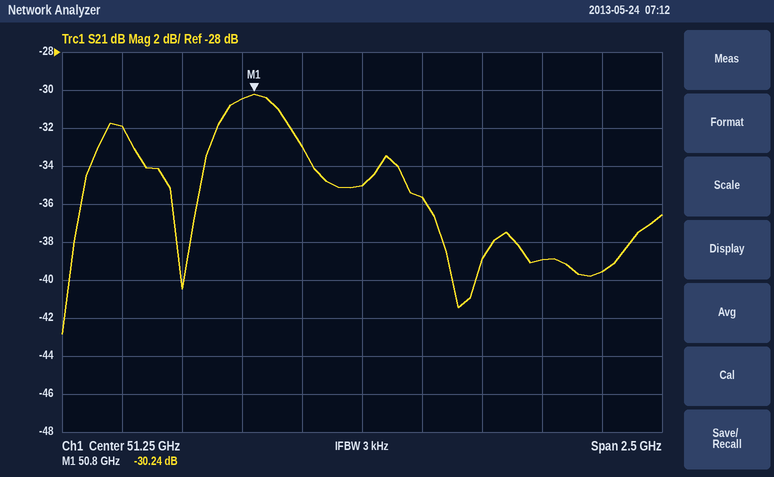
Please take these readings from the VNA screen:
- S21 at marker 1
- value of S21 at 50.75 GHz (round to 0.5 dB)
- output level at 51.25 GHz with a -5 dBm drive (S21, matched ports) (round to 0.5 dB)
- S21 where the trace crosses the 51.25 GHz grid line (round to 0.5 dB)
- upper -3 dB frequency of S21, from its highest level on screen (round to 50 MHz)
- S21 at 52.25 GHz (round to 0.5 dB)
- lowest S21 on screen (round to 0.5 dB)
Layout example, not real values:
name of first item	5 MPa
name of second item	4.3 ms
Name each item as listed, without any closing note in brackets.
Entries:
S21 at marker 1	-30.24 dB
value of S21 at 50.75 GHz	-30.5 dB
output level at 51.25 GHz with a -5 dBm drive (S21, matched ports)	-40.0 dBm
S21 where the trace crosses the 51.25 GHz grid line	-35.0 dB
upper -3 dB frequency of S21, from its highest level on screen	51.00 GHz
S21 at 52.25 GHz	-39.5 dB
lowest S21 on screen	-43.0 dB
